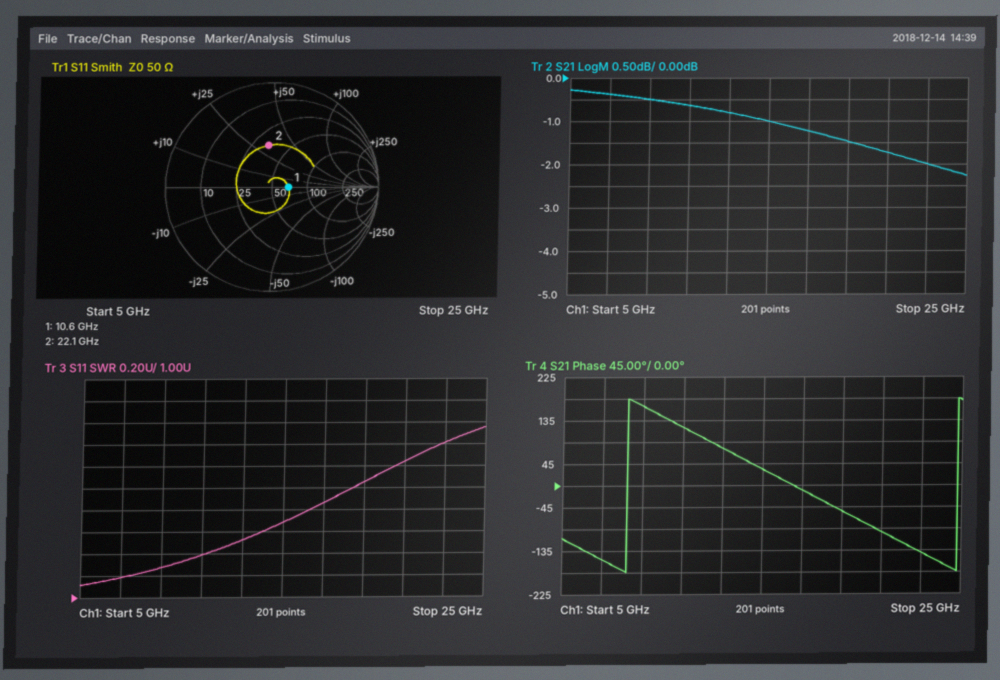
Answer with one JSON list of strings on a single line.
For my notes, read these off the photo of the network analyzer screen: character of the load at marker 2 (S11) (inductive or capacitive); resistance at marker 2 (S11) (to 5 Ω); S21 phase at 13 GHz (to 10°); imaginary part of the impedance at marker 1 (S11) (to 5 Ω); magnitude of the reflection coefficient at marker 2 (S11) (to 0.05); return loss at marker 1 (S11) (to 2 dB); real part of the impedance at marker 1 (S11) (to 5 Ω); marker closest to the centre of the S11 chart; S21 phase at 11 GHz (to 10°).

["inductive", "35 Ω", "80°", "0 Ω", "0.40", "16 dB", "70 Ω", "marker 1", "120°"]
